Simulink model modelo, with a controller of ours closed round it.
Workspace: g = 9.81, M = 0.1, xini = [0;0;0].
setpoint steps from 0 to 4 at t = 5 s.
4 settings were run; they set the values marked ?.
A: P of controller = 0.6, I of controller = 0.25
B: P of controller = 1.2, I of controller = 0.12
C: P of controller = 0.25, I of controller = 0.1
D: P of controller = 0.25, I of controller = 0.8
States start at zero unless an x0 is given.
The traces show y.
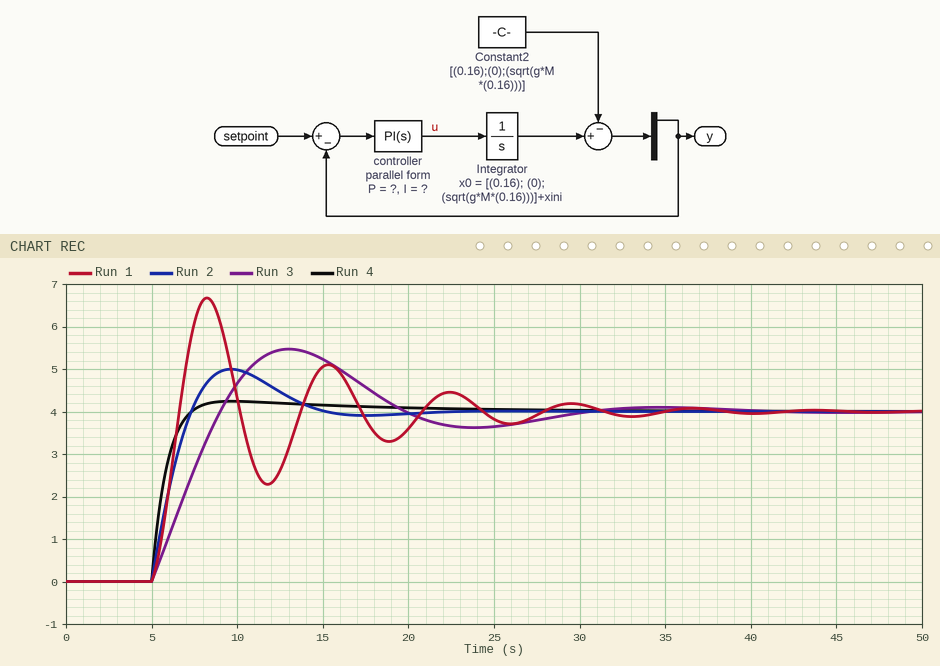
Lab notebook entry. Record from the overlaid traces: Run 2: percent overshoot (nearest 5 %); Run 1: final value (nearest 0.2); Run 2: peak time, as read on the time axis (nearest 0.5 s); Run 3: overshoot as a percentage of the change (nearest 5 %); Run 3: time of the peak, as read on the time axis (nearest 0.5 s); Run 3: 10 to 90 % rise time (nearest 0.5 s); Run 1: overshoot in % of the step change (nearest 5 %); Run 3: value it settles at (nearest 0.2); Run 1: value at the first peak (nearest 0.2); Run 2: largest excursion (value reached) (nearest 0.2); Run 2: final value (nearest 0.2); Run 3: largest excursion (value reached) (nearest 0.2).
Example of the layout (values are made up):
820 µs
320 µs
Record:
25 %
4.0
9.5 s
35 %
13.0 s
3.0 s
65 %
4.0
6.6
5.0
4.0
5.4
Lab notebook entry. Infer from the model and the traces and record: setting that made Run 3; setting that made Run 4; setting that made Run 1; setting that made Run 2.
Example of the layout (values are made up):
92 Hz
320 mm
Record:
C
B
D
A
